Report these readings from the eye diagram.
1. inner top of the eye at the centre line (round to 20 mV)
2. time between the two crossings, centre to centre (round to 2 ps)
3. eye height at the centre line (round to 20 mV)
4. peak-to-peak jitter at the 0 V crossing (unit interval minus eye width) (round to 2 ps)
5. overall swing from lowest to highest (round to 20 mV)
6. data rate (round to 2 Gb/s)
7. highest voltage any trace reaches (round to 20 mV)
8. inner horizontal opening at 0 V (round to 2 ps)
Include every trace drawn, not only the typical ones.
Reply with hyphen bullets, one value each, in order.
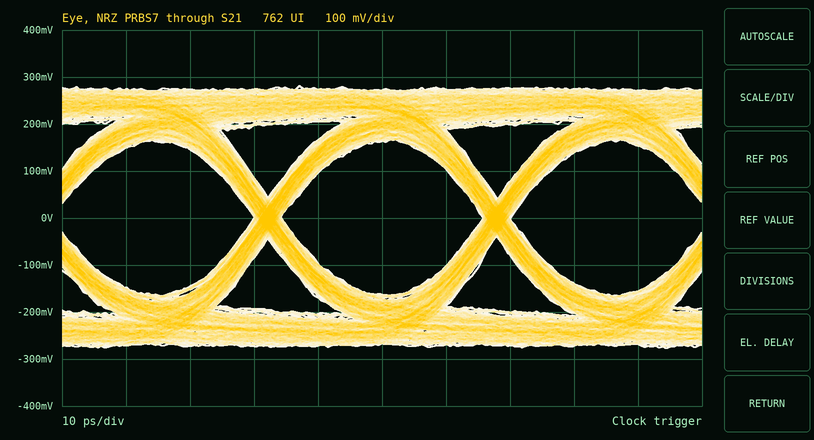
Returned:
- 160 mV
- 36 ps
- 320 mV
- 4 ps
- 560 mV
- 28 Gb/s
- 280 mV
- 32 ps
